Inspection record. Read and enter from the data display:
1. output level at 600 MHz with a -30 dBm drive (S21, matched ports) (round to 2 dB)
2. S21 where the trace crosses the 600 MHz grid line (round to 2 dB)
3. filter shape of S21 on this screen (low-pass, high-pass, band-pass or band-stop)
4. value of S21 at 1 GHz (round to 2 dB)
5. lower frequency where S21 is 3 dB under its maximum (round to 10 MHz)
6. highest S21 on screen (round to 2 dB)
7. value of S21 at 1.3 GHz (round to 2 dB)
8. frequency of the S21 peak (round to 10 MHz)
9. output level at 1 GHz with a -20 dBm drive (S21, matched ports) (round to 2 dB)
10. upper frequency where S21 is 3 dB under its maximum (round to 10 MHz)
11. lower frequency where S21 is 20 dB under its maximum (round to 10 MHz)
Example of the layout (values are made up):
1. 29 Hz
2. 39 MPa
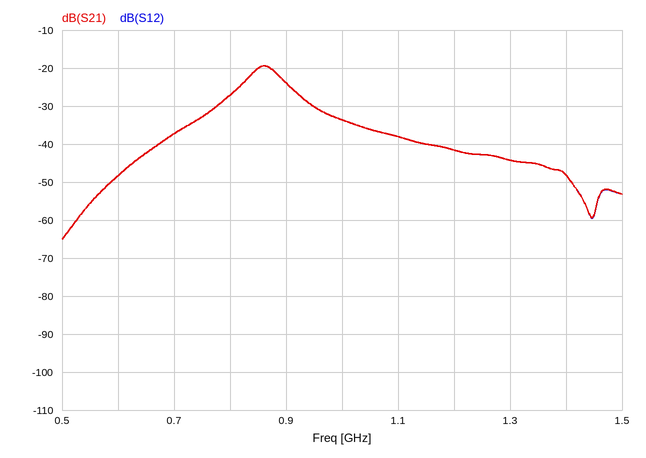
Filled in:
1. -78 dBm
2. -48 dB
3. band-pass
4. -34 dB
5. 830 MHz
6. -20 dB
7. -44 dB
8. 860 MHz
9. -54 dBm
10. 890 MHz
11. 680 MHz
